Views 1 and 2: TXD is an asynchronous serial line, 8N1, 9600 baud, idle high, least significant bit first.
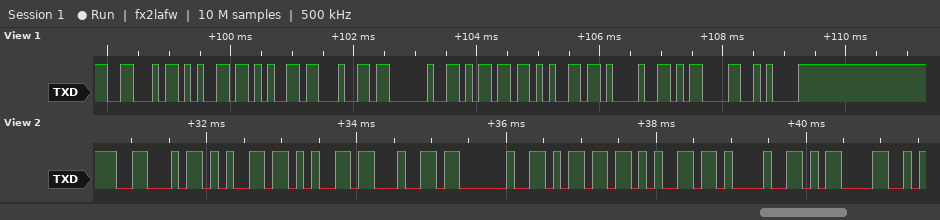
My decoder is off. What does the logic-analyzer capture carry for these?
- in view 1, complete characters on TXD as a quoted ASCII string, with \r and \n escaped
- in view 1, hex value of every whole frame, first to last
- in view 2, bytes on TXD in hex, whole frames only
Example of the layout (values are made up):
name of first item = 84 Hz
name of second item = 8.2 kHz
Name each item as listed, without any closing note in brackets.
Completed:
in view 1, complete characters on TXD as a quoted ASCII string, with \r and \n escaped = "Feed me!\r\n"
in view 1, hex value of every whole frame, first to last = 0x46 0x65 0x65 0x64 0x20 0x6D 0x65 0x21 0x0D 0x0A
in view 2, bytes on TXD in hex, whole frames only = 0x46 0x65 0x65 0x64 0x20 0x6D 0x65 0x21 0x0D
